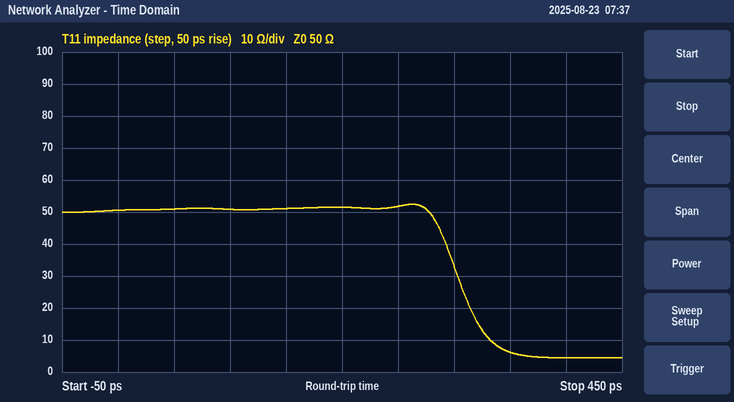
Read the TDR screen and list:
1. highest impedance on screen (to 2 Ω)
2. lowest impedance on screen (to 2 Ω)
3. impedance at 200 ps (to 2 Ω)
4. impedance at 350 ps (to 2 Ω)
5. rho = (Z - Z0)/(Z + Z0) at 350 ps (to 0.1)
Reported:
52 Ω
4 Ω
52 Ω
6 Ω
-0.8
